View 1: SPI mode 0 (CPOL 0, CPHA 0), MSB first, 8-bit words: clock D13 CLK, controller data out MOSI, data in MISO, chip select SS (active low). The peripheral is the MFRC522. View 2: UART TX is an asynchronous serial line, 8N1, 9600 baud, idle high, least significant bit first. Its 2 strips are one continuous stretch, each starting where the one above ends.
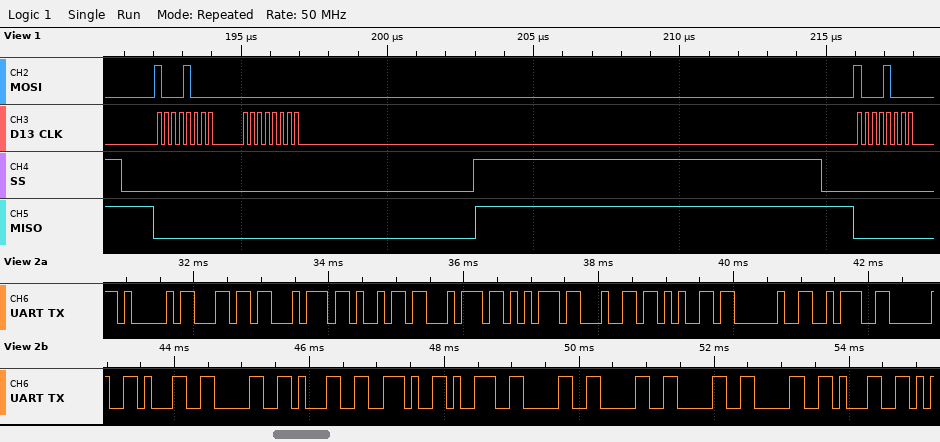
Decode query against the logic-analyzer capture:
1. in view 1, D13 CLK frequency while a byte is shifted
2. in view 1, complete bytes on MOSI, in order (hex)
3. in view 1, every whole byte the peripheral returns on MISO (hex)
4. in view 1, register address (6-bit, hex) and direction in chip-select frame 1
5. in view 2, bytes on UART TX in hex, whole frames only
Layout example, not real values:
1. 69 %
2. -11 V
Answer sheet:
1. 4 MHz
2. 88 00 88
3. 00 00 00
4. 0x04 read
5. 0x41 0x6C 0x74 0x69 0x74 0x75 0x64 0x65 0x20 0x3A 0x20 0x31 0x30 0x31 0x2E 0x39 0x30 0x30 0x30 0x30 0x31
